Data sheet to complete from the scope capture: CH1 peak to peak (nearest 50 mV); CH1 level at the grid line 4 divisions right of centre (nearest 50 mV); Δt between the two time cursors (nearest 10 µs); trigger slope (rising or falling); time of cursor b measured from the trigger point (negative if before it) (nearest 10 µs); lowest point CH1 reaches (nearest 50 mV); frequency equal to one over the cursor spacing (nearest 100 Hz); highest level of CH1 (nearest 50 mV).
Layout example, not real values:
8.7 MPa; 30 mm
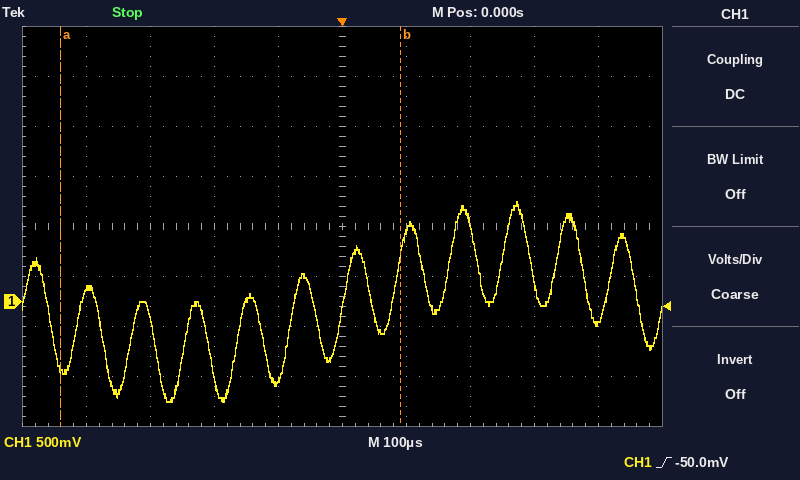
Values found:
2.00 V; -200 mV; 530 µs; rising; +90 µs; -1.00 V; 1.9 kHz; 1.00 V
